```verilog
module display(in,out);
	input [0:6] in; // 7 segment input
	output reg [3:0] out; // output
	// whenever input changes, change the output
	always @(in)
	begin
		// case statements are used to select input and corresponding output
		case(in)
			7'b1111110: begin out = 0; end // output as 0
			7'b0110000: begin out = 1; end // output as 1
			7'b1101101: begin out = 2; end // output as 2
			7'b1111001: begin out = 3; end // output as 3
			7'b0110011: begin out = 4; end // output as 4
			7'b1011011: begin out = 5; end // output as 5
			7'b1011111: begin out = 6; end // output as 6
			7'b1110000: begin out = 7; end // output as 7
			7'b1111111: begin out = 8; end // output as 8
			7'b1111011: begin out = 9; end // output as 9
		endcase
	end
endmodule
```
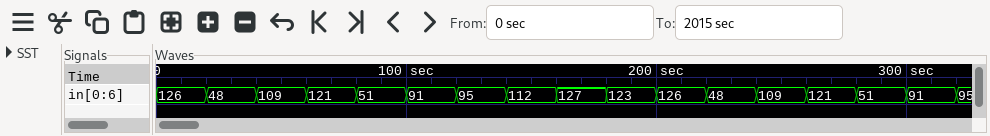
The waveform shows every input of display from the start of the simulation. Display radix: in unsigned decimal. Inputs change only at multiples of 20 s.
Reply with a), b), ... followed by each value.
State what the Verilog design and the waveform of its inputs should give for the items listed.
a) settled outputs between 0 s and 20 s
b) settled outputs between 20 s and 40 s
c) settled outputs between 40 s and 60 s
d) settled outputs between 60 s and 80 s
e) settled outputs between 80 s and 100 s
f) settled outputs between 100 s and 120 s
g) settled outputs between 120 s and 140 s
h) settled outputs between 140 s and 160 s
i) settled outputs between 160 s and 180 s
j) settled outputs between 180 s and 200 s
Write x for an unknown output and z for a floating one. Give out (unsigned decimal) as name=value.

a) out=0
b) out=1
c) out=2
d) out=3
e) out=4
f) out=5
g) out=6
h) out=7
i) out=8
j) out=9
